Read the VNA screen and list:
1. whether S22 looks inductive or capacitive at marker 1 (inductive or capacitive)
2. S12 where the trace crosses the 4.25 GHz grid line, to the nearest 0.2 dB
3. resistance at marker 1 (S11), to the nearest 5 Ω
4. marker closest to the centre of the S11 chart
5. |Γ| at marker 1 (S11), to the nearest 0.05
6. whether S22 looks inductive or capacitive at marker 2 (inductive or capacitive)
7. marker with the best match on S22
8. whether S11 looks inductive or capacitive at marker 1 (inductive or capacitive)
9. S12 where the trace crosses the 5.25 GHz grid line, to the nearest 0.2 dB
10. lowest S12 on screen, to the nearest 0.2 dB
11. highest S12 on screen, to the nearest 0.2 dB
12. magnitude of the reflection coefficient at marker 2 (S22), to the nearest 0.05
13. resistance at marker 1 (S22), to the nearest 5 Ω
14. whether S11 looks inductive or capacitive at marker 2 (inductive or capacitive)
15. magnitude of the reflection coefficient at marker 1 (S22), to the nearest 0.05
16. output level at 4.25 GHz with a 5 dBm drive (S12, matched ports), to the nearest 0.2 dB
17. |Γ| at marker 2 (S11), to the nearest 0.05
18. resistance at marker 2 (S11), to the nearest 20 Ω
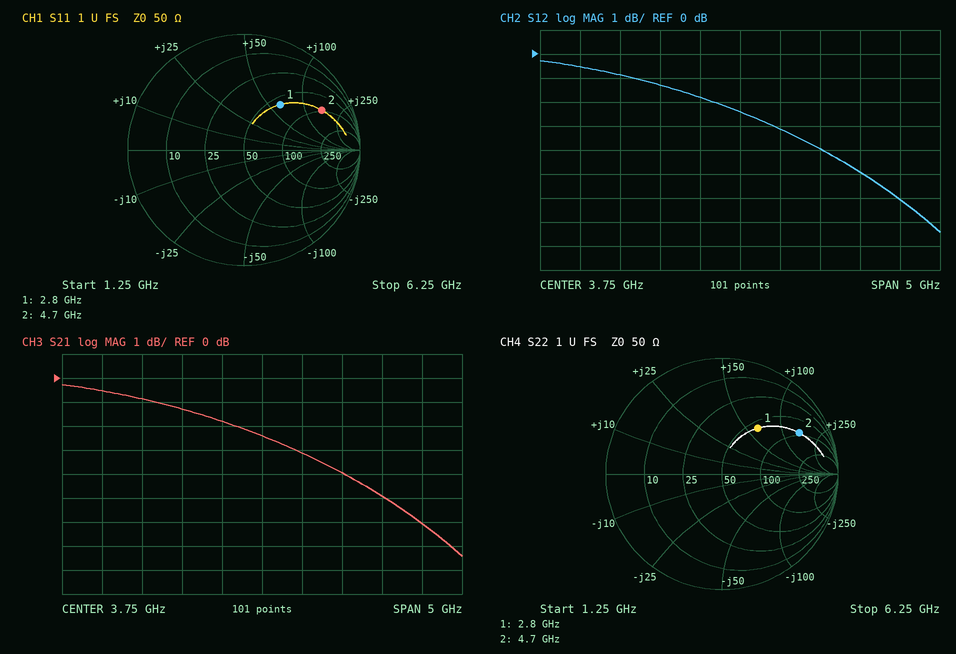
inductive
-3.2 dB
60 Ω
marker 1
0.50
inductive
marker 1
inductive
-5.0 dB
-7.4 dB
-0.2 dB
0.75
60 Ω
inductive
0.50
1.8 dBm
0.75
100 Ω
